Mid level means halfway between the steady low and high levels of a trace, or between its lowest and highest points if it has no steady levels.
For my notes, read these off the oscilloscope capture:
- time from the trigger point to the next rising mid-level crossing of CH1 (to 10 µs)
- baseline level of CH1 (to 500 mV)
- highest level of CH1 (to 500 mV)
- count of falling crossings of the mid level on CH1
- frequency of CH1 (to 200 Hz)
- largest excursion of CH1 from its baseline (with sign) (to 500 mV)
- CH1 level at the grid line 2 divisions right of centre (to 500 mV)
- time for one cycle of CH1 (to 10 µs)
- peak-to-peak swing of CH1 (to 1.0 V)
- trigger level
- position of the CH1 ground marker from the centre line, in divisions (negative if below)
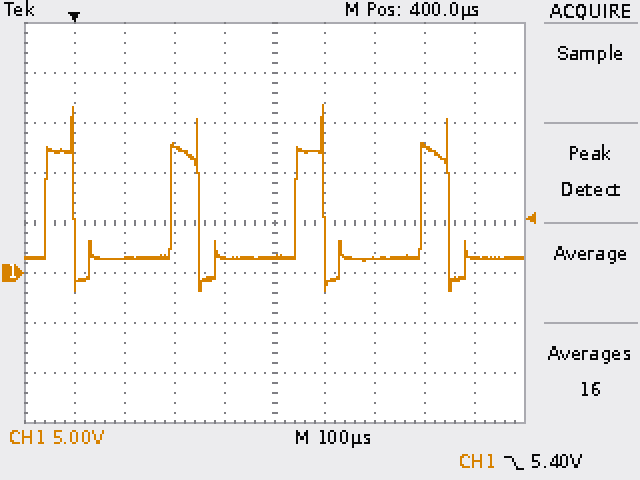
190 µs
1.5 V
17.0 V
4
4.0 kHz
+15.5 V
1.5 V
250 µs
19.0 V
5.40 V
-1.0 div
